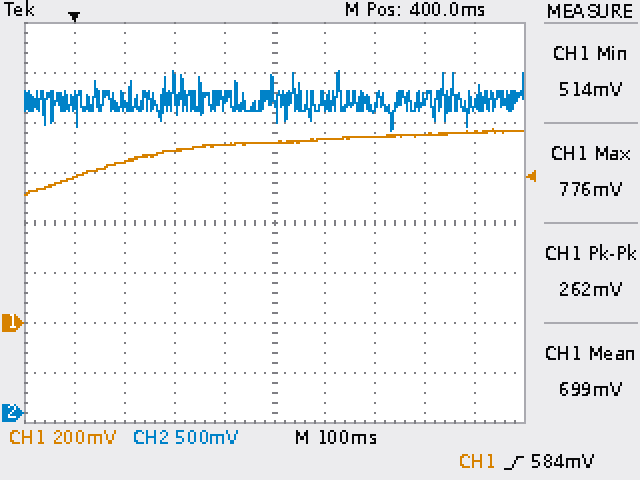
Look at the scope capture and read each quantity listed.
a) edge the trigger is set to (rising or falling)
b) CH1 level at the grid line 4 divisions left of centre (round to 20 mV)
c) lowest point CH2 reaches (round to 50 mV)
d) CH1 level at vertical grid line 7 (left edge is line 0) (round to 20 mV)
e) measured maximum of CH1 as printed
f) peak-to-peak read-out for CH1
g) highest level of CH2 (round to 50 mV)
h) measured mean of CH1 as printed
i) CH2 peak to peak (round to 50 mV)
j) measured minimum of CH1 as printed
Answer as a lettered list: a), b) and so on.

a) rising
b) 580 mV
c) 2.80 V
d) 740 mV
e) 776 mV
f) 262 mV
g) 3.40 V
h) 699 mV
i) 600 mV
j) 514 mV
